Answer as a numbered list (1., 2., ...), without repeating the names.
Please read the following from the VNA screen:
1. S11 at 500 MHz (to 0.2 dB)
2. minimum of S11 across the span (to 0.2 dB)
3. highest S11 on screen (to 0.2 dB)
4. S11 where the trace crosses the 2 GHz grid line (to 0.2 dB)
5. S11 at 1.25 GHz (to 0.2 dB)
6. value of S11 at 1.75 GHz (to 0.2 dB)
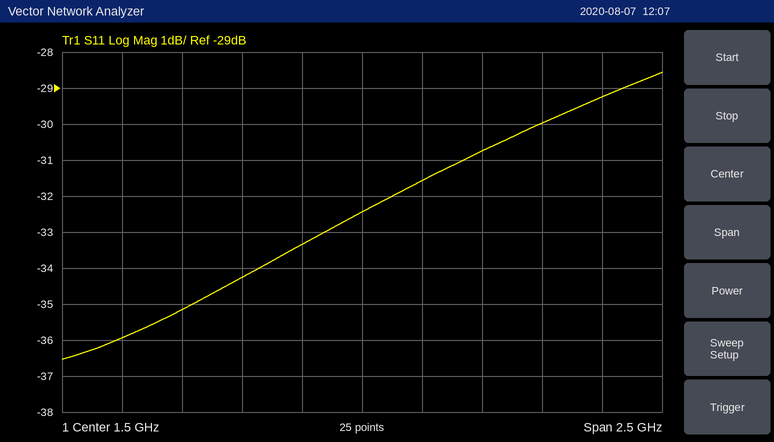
1. -36.0 dB
2. -36.6 dB
3. -28.6 dB
4. -30.8 dB
5. -33.4 dB
6. -31.6 dB
